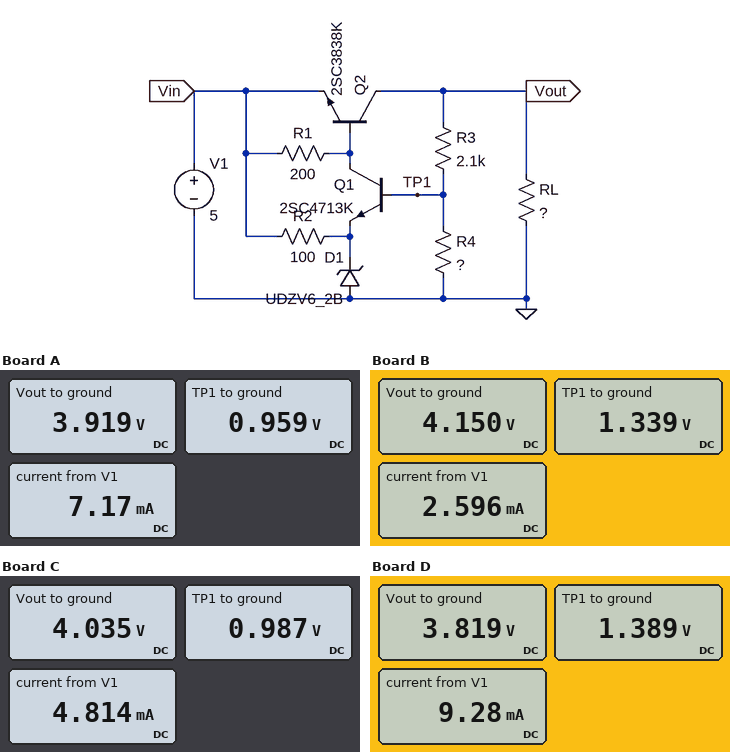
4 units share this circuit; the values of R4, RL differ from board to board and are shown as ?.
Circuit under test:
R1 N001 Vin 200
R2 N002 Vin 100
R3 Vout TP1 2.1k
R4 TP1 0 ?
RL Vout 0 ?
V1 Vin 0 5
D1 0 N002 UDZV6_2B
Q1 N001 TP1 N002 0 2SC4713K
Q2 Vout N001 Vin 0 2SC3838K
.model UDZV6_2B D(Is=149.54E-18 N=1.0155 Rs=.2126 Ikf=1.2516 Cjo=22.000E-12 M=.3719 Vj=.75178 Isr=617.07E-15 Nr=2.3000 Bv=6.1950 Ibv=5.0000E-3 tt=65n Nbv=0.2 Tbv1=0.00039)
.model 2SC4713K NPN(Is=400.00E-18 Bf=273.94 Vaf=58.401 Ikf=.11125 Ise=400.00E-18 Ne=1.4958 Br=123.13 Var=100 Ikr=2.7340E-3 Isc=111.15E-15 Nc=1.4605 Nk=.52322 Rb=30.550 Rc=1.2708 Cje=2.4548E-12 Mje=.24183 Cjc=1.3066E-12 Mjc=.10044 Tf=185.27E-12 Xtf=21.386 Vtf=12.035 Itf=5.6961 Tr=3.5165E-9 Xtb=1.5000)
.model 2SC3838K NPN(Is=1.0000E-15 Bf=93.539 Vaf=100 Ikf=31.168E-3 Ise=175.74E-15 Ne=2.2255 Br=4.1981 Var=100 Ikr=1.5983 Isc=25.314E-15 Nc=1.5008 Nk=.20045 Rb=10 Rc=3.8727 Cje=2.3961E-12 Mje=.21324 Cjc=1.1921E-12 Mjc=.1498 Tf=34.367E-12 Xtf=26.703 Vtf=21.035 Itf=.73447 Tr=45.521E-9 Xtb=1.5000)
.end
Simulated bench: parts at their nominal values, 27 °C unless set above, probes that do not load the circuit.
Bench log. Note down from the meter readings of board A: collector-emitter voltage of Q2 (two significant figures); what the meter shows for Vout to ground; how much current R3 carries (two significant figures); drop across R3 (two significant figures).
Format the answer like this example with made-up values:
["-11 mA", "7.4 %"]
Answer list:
["-1.1 V", "3.919 V", "1.4 mA", "3.0 V"]
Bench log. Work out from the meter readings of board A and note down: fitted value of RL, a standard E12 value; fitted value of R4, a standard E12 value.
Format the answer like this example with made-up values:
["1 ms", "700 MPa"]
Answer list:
["680 Ω", "680 Ω"]
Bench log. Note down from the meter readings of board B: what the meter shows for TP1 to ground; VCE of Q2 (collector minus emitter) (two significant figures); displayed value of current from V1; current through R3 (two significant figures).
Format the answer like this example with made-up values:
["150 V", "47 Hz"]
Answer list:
["1.339 V", "-850 mV", "2.596 mA", "1.3 mA"]
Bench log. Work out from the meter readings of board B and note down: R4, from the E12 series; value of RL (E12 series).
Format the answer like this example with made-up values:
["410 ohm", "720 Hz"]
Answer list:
["1 kΩ", "3.3 kΩ"]
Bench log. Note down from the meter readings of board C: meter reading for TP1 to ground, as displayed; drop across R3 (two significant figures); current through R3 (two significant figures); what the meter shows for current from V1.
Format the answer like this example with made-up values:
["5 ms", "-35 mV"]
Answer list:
["0.987 V", "3.0 V", "1.5 mA", "4.814 mA"]
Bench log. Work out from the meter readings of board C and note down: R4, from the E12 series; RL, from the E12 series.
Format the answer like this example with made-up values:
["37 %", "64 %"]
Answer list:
["680 Ω", "1.2 kΩ"]
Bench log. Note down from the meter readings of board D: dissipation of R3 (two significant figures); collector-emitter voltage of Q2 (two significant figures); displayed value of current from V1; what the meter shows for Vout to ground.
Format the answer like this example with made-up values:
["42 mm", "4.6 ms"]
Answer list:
["2.8 mW", "-1.2 V", "9.28 mA", "3.819 V"]
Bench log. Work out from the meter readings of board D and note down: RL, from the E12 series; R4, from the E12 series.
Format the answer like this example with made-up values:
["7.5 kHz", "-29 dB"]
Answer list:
["470 Ω", "1.2 kΩ"]
